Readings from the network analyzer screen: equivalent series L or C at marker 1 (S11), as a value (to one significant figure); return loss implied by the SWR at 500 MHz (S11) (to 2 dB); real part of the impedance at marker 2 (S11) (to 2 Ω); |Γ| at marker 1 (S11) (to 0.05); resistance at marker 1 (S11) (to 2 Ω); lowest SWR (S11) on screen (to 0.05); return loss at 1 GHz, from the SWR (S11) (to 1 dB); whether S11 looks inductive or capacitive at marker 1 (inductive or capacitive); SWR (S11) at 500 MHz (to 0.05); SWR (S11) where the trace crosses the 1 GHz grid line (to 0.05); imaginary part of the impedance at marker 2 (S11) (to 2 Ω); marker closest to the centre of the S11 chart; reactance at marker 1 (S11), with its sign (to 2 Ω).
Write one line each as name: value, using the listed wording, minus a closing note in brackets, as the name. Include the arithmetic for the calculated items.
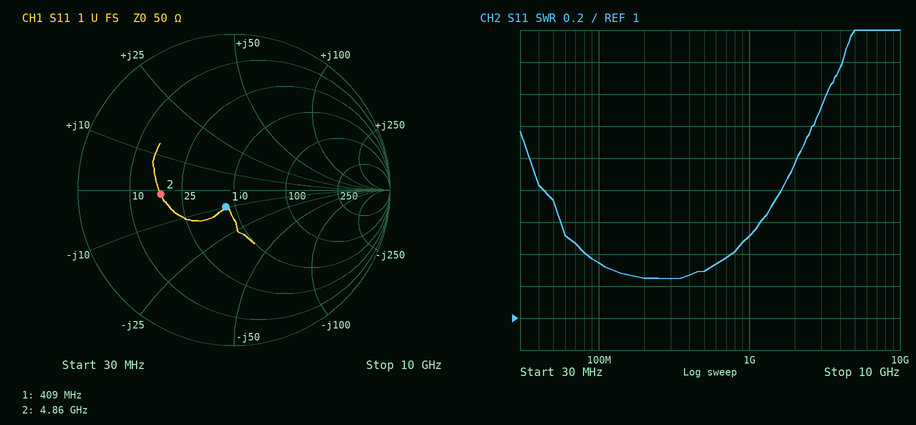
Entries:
equivalent series L or C at marker 1 (S11), as a value: C = 1/(2π × 409 MHz × 10 Ω) ≈ 38.9 pF, so 40 pF to one significant figure
return loss implied by the SWR at 500 MHz (S11): −20 log10((1.3 − 1)/(1.3 + 1)) ≈ 18 dB
real part of the impedance at marker 2 (S11): 18 Ω
|Γ| at marker 1 (S11): 0.10
resistance at marker 1 (S11): 44 Ω
lowest SWR (S11) on screen: 1.25
return loss at 1 GHz, from the SWR (S11): −20 log10((1.5 − 1)/(1.5 + 1)) ≈ 14 dB
whether S11 looks inductive or capacitive at marker 1: capacitive
SWR (S11) at 500 MHz: 1.30
SWR (S11) where the trace crosses the 1 GHz grid line: 1.50
imaginary part of the impedance at marker 2 (S11): -2 Ω
marker closest to the centre of the S11 chart: marker 1
reactance at marker 1 (S11), with its sign: -10 Ω
